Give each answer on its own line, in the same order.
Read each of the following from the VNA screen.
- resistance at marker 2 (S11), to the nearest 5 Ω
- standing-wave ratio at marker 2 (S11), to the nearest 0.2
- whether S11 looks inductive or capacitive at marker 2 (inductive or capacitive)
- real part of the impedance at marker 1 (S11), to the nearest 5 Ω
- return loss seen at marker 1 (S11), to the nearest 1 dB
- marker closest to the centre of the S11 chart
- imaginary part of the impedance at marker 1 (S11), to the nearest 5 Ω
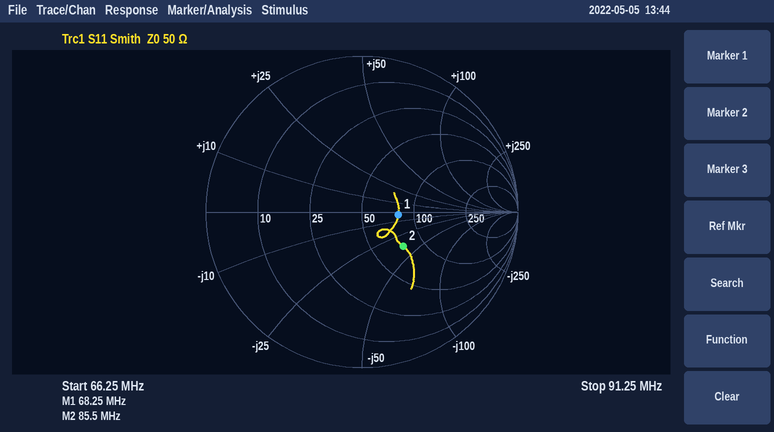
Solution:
75 Ω
2.0
capacitive
80 Ω
13 dB
marker 1
-5 Ω
